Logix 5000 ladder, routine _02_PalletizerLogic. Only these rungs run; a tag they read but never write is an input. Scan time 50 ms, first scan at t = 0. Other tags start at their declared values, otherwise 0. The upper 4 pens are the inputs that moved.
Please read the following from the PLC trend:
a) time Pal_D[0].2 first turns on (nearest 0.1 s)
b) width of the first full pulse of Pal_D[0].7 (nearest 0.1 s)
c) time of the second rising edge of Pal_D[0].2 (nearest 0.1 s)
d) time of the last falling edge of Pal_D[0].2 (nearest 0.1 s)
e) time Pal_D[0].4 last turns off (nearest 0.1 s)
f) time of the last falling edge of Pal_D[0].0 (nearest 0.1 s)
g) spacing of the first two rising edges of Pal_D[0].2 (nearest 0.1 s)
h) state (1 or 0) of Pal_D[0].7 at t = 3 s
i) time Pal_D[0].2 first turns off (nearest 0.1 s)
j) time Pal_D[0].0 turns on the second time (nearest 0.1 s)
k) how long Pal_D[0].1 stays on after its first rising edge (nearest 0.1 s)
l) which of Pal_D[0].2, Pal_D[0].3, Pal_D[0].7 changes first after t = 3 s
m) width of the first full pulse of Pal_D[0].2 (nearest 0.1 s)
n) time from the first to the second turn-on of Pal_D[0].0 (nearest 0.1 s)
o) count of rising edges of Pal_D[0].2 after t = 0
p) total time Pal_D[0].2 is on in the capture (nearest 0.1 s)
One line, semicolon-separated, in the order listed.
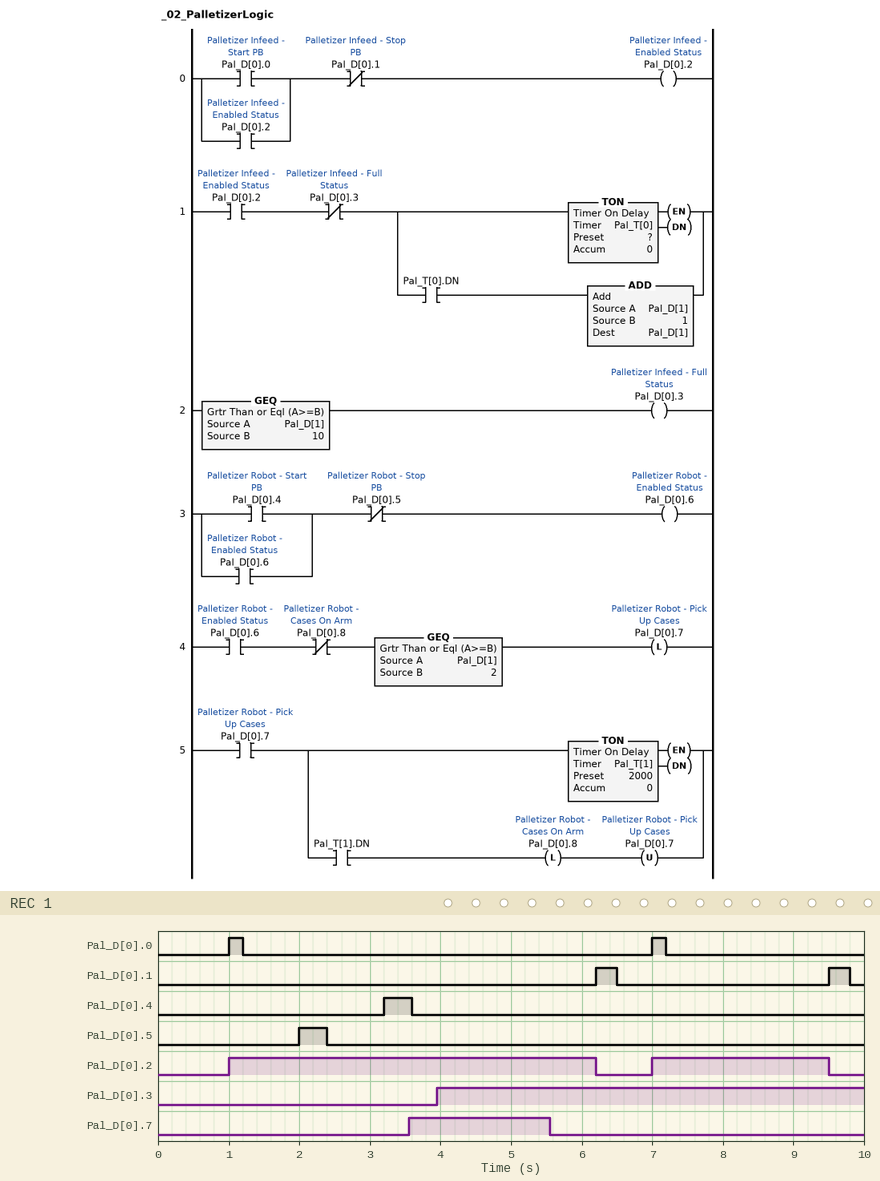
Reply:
1.0 s; 2.0 s; 7.0 s; 9.5 s; 3.6 s; 7.2 s; 6.0 s; 0; 6.2 s; 7.0 s; 0.3 s; Pal_D[0].7; 5.2 s; 6.0 s; 2; 7.7 s
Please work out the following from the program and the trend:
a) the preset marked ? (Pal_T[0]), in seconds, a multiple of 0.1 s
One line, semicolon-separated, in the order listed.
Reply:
2.5 s
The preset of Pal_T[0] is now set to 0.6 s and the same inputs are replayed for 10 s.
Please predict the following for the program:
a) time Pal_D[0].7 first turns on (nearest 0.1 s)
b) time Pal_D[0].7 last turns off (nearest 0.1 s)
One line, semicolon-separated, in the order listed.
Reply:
3.2 s; 5.2 s
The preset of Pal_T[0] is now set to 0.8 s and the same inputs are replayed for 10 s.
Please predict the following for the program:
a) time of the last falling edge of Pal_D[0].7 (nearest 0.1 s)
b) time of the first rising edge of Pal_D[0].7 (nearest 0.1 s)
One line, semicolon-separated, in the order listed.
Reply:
5.2 s; 3.2 s
